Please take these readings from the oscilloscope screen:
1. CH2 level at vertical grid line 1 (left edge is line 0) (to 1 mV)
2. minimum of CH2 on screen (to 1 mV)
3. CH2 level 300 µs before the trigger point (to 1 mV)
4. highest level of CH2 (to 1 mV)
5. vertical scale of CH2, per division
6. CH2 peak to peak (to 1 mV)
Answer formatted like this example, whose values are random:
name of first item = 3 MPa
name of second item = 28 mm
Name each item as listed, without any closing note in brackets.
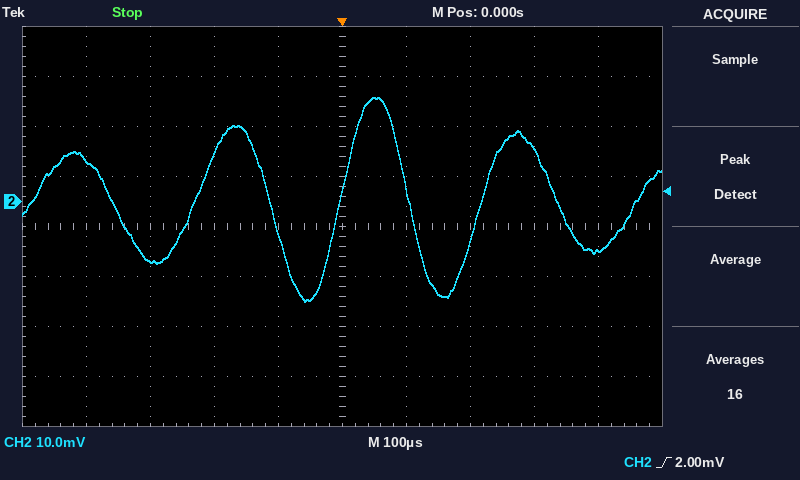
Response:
CH2 level at vertical grid line 1 (left edge is line 0) = 8 mV
minimum of CH2 on screen = -20 mV
CH2 level 300 µs before the trigger point = -12 mV
highest level of CH2 = 21 mV
vertical scale of CH2, per division = 10 mV
CH2 peak to peak = 41 mV
